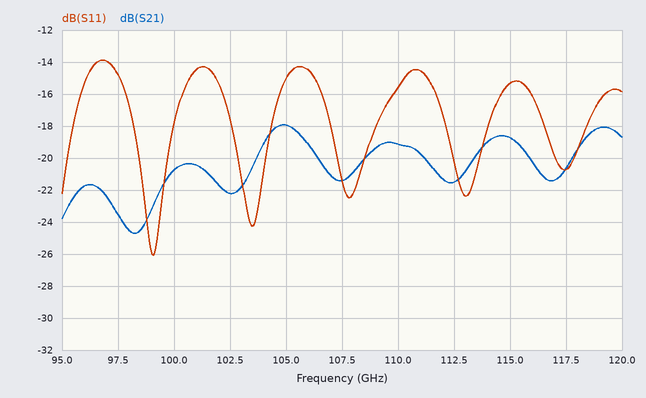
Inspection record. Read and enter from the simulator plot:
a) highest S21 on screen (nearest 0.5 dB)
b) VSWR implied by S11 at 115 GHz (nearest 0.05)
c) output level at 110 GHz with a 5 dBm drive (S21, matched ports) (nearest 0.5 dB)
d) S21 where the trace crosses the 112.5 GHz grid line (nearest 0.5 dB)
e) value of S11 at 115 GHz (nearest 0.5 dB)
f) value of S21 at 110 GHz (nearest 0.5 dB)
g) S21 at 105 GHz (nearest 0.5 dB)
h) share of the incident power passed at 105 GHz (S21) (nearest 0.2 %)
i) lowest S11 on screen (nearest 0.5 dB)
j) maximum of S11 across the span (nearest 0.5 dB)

-18.0 dB
1.40
-14.0 dBm
-21.5 dB
-15.5 dB
-19.0 dB
-18.0 dB
1.6 %
-26.0 dB
-14.0 dB
